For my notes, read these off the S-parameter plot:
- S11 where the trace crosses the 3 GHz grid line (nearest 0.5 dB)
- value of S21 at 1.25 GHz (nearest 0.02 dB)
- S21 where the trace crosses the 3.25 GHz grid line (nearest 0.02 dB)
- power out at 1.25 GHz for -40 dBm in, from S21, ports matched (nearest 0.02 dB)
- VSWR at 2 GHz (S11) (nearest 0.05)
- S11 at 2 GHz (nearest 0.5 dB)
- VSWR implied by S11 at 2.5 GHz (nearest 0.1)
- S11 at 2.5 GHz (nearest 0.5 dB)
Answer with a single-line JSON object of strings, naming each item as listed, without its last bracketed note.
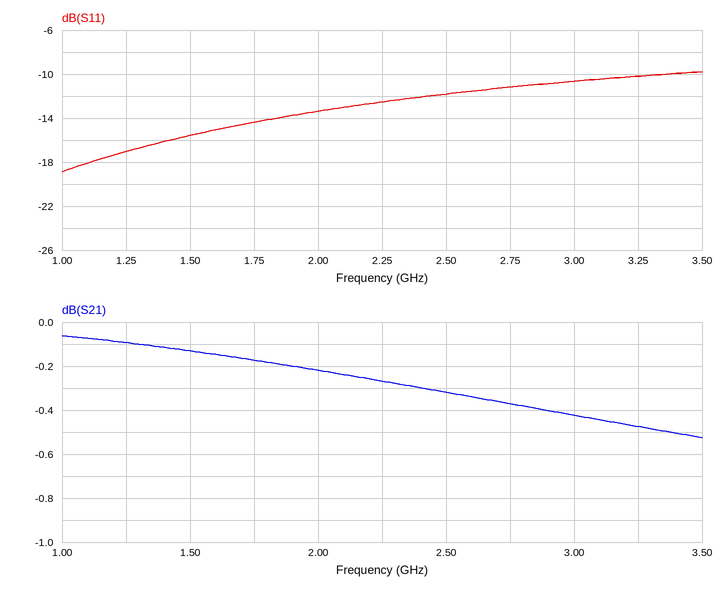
{"S11 where the trace crosses the 3 GHz grid line": "-10.5 dB", "value of S21 at 1.25 GHz": "-0.10 dB", "S21 where the trace crosses the 3.25 GHz grid line": "-0.48 dB", "power out at 1.25 GHz for -40 dBm in, from S21, ports matched": "-40.10 dBm", "VSWR at 2 GHz (S11)": "1.55", "S11 at 2 GHz": "-13.5 dB", "VSWR implied by S11 at 2.5 GHz": "1.7", "S11 at 2.5 GHz": "-12.0 dB"}
